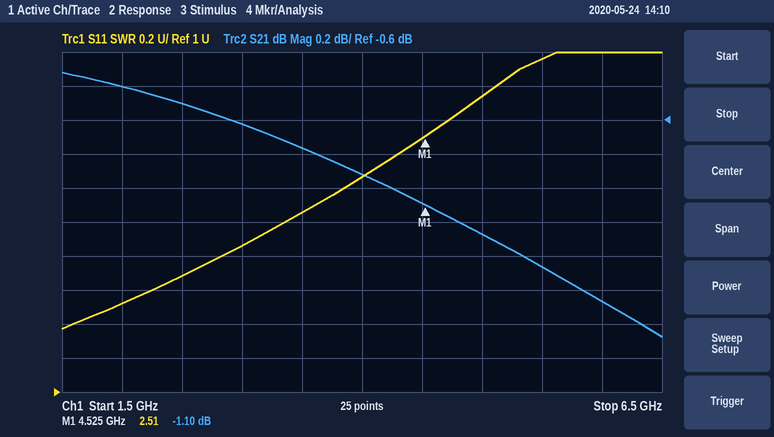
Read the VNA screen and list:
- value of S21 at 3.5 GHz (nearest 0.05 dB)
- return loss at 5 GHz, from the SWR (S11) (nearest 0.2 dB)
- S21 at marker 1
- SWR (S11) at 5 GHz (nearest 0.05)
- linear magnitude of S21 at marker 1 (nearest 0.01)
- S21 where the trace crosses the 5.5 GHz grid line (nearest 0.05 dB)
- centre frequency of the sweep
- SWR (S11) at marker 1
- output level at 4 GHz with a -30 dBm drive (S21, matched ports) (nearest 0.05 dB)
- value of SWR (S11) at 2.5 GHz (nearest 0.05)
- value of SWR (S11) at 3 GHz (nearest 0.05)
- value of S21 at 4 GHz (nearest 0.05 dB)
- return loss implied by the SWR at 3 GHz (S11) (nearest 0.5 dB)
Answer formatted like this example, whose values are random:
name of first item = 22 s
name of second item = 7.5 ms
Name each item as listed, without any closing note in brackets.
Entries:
value of S21 at 3.5 GHz = -0.75 dB
return loss at 5 GHz, from the SWR (S11) = 6.6 dB
S21 at marker 1 = -1.10 dB
SWR (S11) at 5 GHz = 2.75
linear magnitude of S21 at marker 1 = 0.88
S21 where the trace crosses the 5.5 GHz grid line = -1.45 dB
centre frequency of the sweep = 4 GHz
SWR (S11) at marker 1 = 2.51
output level at 4 GHz with a -30 dBm drive (S21, matched ports) = -30.90 dBm
value of SWR (S11) at 2.5 GHz = 1.70
value of SWR (S11) at 3 GHz = 1.85
value of S21 at 4 GHz = -0.90 dB
return loss implied by the SWR at 3 GHz (S11) = 10.5 dB
